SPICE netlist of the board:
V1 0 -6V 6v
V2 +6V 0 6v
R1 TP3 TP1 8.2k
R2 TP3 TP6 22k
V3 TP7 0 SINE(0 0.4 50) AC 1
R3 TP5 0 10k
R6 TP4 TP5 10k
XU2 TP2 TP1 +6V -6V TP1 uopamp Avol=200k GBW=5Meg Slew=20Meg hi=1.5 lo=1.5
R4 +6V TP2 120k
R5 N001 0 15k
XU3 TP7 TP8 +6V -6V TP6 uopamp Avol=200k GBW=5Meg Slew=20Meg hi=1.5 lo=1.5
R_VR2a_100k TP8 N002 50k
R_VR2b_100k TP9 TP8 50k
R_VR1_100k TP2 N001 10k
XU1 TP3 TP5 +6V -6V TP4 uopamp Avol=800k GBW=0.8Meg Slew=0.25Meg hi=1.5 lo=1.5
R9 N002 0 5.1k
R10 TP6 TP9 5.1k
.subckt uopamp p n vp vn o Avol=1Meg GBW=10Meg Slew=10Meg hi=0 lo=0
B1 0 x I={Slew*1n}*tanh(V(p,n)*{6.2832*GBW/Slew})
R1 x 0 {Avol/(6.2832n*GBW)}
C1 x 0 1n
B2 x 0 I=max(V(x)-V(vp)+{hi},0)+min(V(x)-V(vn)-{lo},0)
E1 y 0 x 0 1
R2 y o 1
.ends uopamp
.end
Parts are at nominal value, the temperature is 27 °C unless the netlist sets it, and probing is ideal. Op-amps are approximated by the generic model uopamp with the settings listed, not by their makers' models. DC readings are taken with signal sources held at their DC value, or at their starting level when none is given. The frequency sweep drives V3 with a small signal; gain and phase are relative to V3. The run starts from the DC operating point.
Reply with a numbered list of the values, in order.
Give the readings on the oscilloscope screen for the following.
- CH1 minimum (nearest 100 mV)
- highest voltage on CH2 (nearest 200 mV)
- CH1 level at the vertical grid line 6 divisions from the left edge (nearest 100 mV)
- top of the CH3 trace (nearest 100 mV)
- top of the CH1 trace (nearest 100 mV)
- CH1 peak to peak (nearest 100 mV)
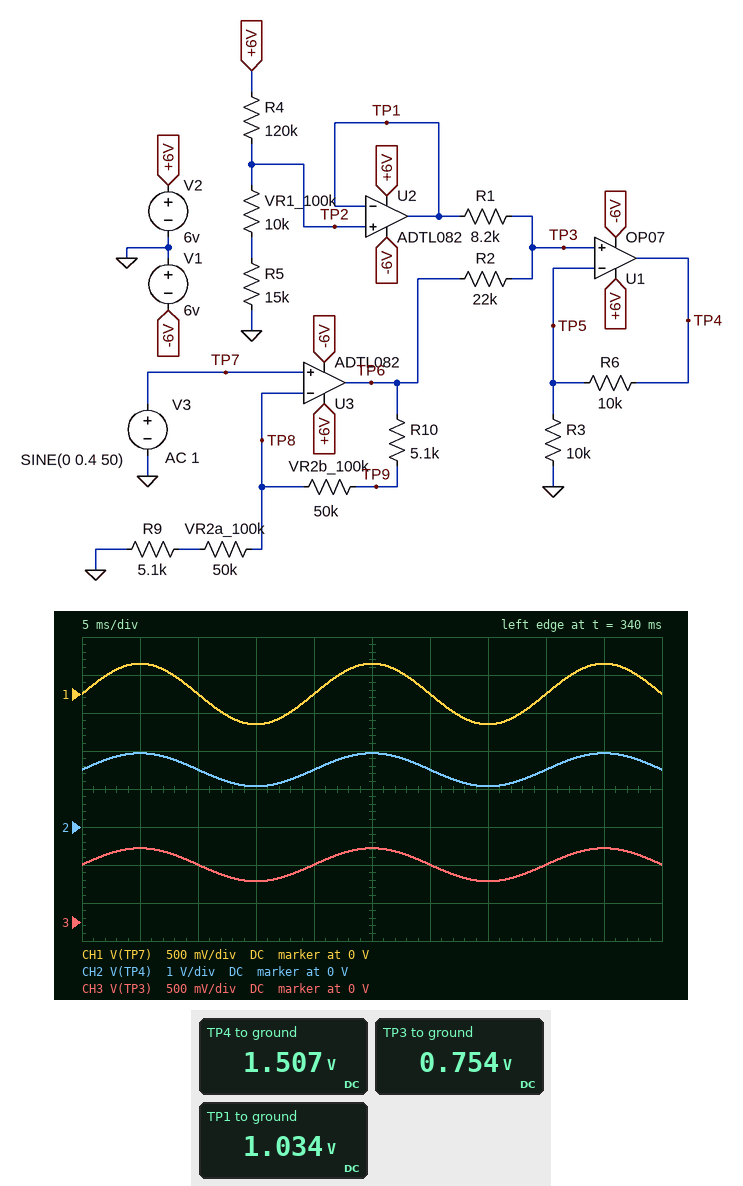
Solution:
1. -400 mV
2. 2.0 V
3. 0 V
4. 1.0 V
5. 400 mV
6. 800 mV
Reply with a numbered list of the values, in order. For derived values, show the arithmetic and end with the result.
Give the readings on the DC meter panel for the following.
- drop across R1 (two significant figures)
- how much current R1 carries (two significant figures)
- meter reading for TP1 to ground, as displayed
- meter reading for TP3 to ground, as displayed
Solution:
1. 1.034 V - 754 mV = 280 mV
2. (1.034 V - 754 mV) / 8.2 kΩ = 34 µA
3. 1.034 V
4. 0.754 V
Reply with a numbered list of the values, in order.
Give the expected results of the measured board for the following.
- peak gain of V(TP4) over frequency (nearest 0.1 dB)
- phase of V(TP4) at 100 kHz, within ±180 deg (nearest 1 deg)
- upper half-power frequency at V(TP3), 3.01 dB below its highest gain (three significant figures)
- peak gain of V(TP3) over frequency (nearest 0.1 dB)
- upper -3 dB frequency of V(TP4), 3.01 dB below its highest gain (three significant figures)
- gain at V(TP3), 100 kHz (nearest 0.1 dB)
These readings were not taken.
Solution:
1. 0.7 dB
2. -16 deg
3. 2.50 MHz
4. -5.3 dB
5. 390 kHz
6. -5.3 dB
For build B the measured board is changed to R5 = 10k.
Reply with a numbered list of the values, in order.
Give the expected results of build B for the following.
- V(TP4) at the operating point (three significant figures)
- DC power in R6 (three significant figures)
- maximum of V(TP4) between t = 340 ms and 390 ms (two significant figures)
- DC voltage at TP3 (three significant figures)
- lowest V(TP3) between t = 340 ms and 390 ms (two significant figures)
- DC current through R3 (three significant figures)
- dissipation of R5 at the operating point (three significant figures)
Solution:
1. 1.25 V
2. 39.0 µW
3. 1.7 V
4. 624 mV
5. 410 mV
6. 62.4 µA
7. 18.4 µW
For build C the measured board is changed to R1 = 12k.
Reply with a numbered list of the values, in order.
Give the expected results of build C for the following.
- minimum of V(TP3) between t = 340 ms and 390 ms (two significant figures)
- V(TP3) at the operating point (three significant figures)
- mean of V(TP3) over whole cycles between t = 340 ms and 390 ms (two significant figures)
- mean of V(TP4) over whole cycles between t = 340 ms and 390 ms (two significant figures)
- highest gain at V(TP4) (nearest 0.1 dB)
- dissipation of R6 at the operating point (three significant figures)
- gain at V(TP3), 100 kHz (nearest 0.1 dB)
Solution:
1. 390 mV
2. 669 mV
3. 670 mV
4. 1.3 V
5. 3.0 dB
6. 44.8 µW
7. -3.0 dB
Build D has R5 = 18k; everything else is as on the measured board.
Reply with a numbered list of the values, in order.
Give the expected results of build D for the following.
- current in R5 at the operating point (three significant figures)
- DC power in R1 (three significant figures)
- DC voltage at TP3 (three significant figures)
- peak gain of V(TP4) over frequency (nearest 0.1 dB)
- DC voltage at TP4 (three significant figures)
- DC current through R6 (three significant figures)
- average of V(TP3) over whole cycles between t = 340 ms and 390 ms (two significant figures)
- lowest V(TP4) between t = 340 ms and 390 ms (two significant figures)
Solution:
1. 40.5 µA
2. 11.6 µW
3. 827 mV
4. 0.7 dB
5. 1.65 V
6. 82.7 µA
7. 830 mV
8. 1.2 V
